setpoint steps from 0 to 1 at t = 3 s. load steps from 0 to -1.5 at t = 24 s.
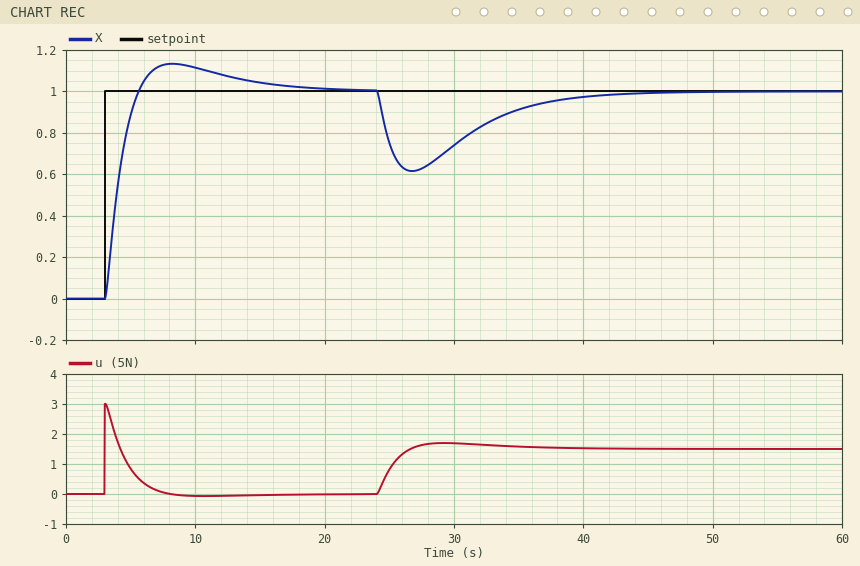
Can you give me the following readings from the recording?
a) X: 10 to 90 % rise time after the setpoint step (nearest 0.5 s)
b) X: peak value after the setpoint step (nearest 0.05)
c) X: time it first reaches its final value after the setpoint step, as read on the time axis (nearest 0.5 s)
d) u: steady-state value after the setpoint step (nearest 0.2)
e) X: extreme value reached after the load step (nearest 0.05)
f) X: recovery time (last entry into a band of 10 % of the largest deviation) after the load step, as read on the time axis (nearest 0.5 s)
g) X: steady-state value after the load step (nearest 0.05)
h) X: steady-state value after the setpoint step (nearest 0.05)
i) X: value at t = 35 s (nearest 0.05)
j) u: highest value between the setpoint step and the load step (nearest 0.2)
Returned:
2.0 s
1.15
5.5 s
0.0
0.60
38.5 s
1.00
1.00
0.90
3.0
